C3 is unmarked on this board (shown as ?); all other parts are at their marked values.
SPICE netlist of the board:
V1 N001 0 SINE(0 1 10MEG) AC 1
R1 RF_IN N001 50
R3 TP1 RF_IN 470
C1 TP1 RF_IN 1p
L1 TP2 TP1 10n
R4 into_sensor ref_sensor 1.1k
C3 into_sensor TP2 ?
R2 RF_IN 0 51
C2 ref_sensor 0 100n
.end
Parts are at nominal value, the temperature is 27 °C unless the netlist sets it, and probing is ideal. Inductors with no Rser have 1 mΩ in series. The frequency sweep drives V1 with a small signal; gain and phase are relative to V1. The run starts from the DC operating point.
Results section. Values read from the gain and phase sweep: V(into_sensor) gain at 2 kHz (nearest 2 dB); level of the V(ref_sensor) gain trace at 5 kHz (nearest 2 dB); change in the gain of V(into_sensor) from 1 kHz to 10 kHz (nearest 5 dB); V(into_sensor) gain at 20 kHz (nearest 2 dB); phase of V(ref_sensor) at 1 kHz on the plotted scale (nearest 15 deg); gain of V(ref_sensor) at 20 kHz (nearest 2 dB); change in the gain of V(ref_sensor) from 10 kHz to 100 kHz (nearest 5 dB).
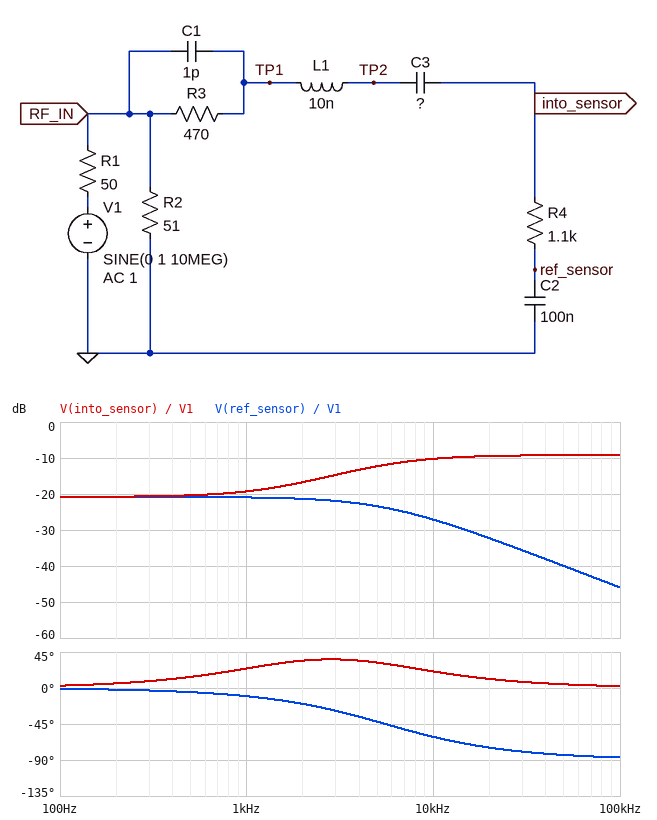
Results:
-16 dB
-24 dB
10 dB
-10 dB
-15 deg
-32 dB
-20 dB
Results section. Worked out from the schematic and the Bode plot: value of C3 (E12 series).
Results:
22 nF
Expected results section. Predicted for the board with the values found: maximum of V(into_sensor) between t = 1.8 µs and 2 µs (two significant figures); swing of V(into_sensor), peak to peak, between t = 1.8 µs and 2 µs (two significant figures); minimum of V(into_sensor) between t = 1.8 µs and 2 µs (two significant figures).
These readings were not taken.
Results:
350 mV
700 mV
-350 mV
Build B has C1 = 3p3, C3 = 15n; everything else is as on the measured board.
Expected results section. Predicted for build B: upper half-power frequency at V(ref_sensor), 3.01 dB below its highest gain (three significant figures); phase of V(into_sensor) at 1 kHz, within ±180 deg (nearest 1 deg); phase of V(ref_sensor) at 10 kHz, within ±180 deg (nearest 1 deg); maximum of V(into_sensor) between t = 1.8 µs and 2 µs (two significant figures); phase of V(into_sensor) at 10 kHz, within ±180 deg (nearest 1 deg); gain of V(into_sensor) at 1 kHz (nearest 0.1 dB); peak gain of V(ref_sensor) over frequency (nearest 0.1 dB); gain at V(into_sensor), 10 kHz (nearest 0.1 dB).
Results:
7.65 kHz
27 deg
-53 deg
350 mV
29 deg
-22.0 dB
-23.6 dB
-11.1 dB
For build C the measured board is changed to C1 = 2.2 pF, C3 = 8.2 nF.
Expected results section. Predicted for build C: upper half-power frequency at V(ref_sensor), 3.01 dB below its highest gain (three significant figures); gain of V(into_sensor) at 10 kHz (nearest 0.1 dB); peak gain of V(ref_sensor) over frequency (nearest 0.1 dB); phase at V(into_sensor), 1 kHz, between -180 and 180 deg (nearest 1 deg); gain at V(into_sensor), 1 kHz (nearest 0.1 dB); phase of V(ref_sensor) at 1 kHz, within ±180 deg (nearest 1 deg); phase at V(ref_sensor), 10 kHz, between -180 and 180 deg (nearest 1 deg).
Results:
13.2 kHz
-13.4 dB
-28.3 dB
30 deg
-26.7 dB
-4 deg
-37 deg
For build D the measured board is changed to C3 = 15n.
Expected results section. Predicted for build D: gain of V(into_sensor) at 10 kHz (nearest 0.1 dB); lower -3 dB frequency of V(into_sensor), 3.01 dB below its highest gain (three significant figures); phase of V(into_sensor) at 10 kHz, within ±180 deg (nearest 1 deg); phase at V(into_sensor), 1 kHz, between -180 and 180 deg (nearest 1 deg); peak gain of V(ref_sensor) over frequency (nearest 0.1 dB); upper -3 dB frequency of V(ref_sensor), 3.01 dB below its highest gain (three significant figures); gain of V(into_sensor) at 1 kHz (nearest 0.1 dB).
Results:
-11.1 dB
7.37 kHz
29 deg
27 deg
-23.6 dB
7.65 kHz
-22.0 dB
